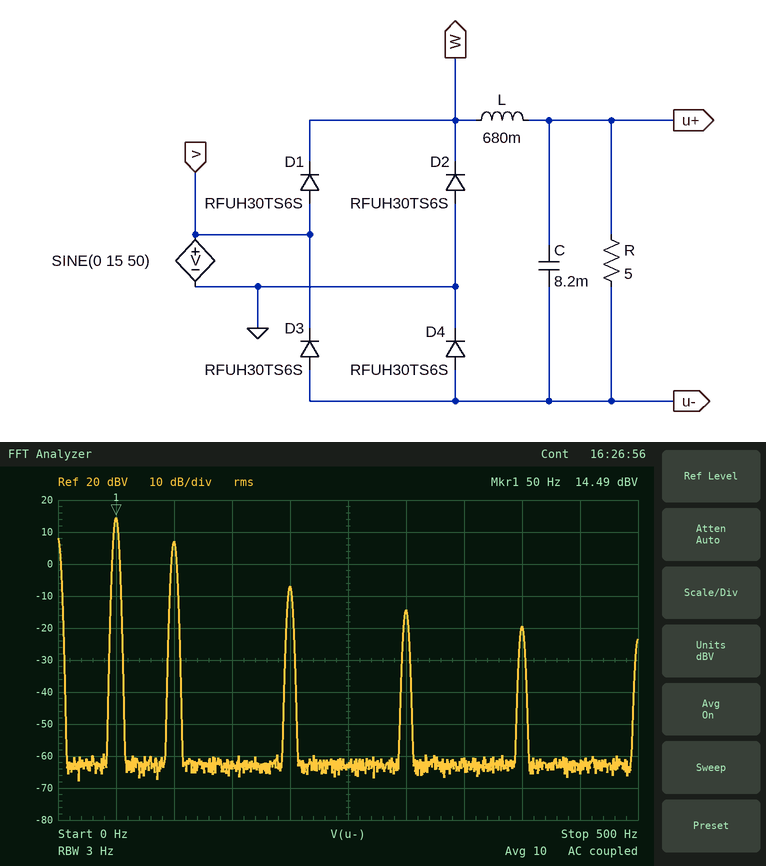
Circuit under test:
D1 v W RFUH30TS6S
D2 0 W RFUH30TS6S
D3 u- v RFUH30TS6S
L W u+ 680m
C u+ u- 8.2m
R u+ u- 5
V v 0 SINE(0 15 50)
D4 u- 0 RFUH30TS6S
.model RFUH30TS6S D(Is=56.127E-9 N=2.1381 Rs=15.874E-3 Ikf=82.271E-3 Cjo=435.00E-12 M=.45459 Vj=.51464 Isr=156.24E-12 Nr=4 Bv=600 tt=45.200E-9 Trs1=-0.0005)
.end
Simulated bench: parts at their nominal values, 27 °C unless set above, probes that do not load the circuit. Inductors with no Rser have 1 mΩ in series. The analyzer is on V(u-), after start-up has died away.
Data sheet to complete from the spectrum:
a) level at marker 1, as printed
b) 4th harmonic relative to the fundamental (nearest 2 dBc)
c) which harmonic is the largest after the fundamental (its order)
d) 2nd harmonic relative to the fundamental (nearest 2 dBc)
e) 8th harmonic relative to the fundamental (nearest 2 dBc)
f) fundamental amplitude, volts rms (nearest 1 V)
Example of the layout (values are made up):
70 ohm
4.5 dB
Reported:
14.49 dBV
-22 dBc
2
-8 dBc
-34 dBc
5 V
